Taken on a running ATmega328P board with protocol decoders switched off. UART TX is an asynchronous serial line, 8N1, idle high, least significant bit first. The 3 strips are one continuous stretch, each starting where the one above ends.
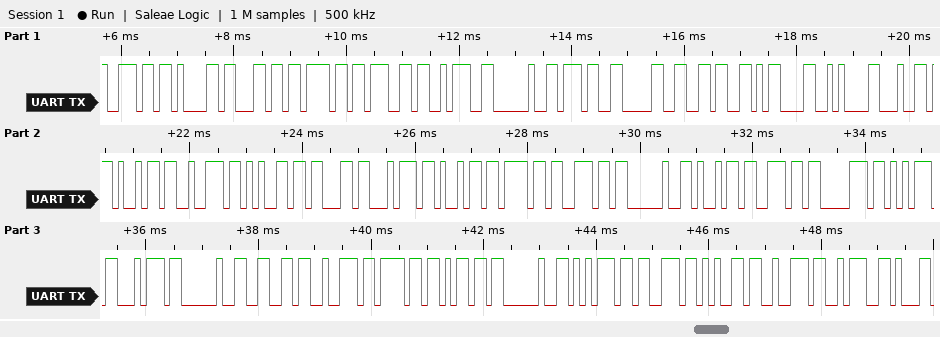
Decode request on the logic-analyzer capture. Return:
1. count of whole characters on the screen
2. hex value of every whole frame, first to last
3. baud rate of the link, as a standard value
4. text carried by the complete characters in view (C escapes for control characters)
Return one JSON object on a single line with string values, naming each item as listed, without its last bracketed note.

{"count of whole characters on the screen": "38", "hex value of every whole frame, first to last": "6E 61 6C 6F 67 3A 20 37 30 36 0D 0A 64 69 72 65 63 74 69 6F 6E 20 69 6E 70 75 74 20 66 72 6F 6D 20 75 73 65 72 3A", "baud rate of the link, as a standard value": "9600 baud", "text carried by the complete characters in view": "\"nalog: 706\\r\\ndirection input from user:\""}
